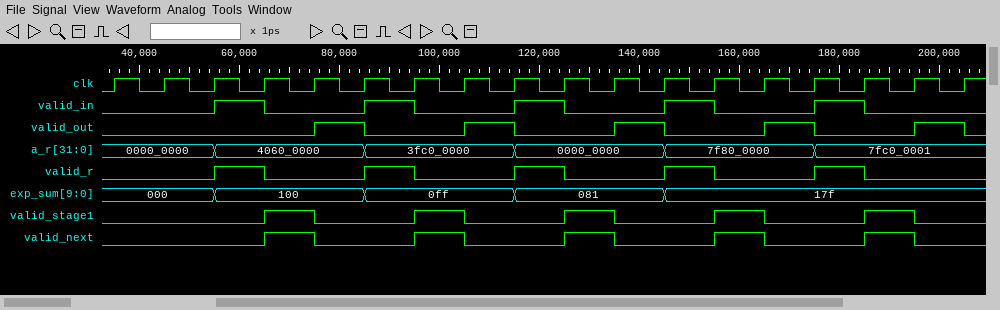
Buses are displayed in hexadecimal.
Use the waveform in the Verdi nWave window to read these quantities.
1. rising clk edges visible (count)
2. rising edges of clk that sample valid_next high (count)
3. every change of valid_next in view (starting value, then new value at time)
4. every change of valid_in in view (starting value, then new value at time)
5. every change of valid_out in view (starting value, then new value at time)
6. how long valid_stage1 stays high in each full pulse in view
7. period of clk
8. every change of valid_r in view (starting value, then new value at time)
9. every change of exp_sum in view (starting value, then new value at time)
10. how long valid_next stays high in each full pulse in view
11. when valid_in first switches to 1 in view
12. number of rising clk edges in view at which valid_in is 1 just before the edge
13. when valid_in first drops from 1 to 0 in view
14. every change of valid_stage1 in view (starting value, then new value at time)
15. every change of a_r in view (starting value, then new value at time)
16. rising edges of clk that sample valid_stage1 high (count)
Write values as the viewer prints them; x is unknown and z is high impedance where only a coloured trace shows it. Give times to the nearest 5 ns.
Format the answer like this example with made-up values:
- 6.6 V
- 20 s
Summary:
- 18
- 5
- 0, 1 at 65 ns, 0 at 75 ns, 1 at 95 ns, 0 at 105 ns, 1 at 125 ns, 0 at 135 ns, 1 at 155 ns, 0 at 165 ns, 1 at 185 ns, 0 at 195 ns
- 0, 1 at 55 ns, 0 at 65 ns, 1 at 85 ns, 0 at 95 ns, 1 at 115 ns, 0 at 125 ns, 1 at 145 ns, 0 at 155 ns, 1 at 175 ns, 0 at 185 ns
- 0, 1 at 75 ns, 0 at 85 ns, 1 at 105 ns, 0 at 115 ns, 1 at 135 ns, 0 at 145 ns, 1 at 165 ns, 0 at 175 ns, 1 at 195 ns, 0 at 205 ns
- 10 ns, 10 ns, 10 ns, 10 ns, 10 ns
- 10 ns
- 0, 1 at 55 ns, 0 at 65 ns, 1 at 85 ns, 0 at 95 ns, 1 at 115 ns, 0 at 125 ns, 1 at 145 ns, 0 at 155 ns, 1 at 175 ns, 0 at 185 ns
- 000, 100 at 55 ns, 0ff at 85 ns, 081 at 115 ns, 17f at 145 ns
- 10 ns, 10 ns, 10 ns, 10 ns, 10 ns
- 55 ns
- 5
- 65 ns
- 0, 1 at 65 ns, 0 at 75 ns, 1 at 95 ns, 0 at 105 ns, 1 at 125 ns, 0 at 135 ns, 1 at 155 ns, 0 at 165 ns, 1 at 185 ns, 0 at 195 ns
- 0000_0000, 4060_0000 at 55 ns, 3fc0_0000 at 85 ns, 0000_0000 at 115 ns, 7f80_0000 at 145 ns, 7fc0_0001 at 175 ns
- 5
